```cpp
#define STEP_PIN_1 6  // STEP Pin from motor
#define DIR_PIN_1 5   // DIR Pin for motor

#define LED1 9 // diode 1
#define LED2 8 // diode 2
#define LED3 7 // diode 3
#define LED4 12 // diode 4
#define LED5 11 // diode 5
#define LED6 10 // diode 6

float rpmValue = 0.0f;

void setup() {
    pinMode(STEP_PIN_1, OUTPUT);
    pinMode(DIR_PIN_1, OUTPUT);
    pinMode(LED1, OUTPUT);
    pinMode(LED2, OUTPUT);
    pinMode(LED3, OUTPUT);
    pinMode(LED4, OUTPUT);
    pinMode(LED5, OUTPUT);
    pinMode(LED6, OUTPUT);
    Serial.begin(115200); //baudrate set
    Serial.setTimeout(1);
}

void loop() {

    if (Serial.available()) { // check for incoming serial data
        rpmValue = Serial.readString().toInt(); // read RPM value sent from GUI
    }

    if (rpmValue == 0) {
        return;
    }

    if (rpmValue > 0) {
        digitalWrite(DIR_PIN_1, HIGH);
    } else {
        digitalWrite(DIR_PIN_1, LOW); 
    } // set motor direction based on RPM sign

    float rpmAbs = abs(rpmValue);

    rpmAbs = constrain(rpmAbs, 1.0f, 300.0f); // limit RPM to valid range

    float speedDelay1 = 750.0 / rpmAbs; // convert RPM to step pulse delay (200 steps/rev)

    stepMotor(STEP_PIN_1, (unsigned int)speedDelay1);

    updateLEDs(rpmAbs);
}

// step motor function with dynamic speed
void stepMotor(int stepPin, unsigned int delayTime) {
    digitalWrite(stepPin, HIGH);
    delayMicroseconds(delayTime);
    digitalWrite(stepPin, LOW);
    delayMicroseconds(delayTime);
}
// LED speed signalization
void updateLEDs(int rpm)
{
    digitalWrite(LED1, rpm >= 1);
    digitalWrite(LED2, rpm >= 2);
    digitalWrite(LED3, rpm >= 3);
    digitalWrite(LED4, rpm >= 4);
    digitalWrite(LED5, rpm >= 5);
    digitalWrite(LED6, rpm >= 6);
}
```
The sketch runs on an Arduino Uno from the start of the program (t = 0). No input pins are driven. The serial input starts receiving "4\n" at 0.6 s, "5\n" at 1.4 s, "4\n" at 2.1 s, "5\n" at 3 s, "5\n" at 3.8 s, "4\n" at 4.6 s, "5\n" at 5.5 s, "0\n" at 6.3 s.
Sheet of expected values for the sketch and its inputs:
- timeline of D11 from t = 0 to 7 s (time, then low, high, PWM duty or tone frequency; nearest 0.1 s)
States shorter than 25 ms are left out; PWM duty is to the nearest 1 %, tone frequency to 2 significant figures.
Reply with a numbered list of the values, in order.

1. 0 s low; 1.4 s high; 2.1 s low; 3 s high; 4.6 s low; 5.5 s high
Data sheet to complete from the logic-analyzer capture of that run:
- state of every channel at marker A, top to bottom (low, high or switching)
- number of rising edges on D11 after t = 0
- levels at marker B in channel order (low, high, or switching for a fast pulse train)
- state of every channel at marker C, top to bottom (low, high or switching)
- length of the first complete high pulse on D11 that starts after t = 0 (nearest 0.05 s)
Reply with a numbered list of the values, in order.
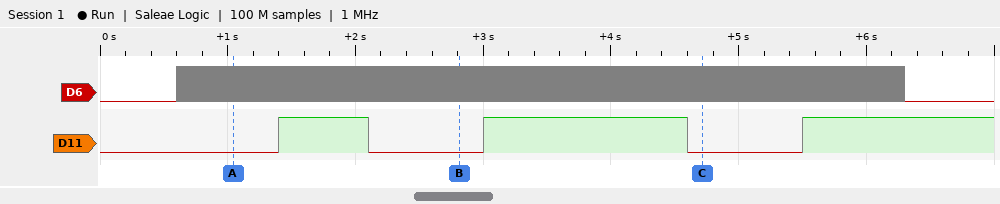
1. D6 switching, D11 low
2. 3
3. D6 switching, D11 low
4. D6 switching, D11 low
5. 0.70 s
